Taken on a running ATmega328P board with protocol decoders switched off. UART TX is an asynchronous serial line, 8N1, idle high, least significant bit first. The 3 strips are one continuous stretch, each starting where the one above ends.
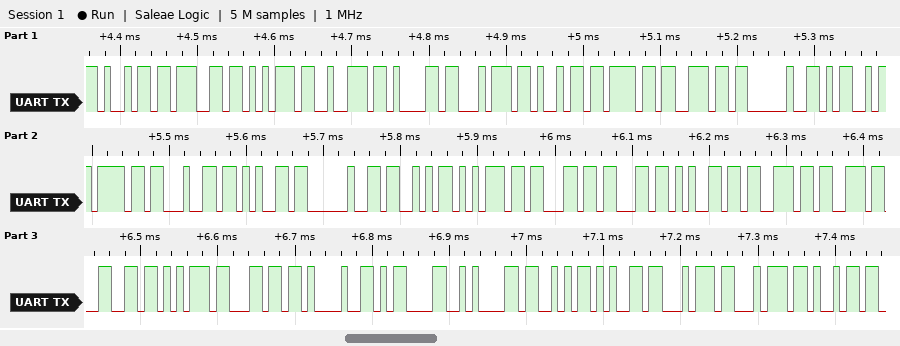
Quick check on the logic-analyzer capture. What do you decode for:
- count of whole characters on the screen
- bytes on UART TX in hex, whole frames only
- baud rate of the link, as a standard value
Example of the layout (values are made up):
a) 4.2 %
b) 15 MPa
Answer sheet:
a) 33
b) 0x69 0x67 0x75 0x72 0x61 0x74 0x69 0x6F 0x6E 0x20 0x4D 0x6F 0x64 0x65 0x20 0x53 0x75 0x63 0x63 0x65 0x73 0x73 0x66 0x75 0x6C 0x21 0x0D 0x0A 0x53 0x65 0x74 0x74 0x69
c) 115200 baud
